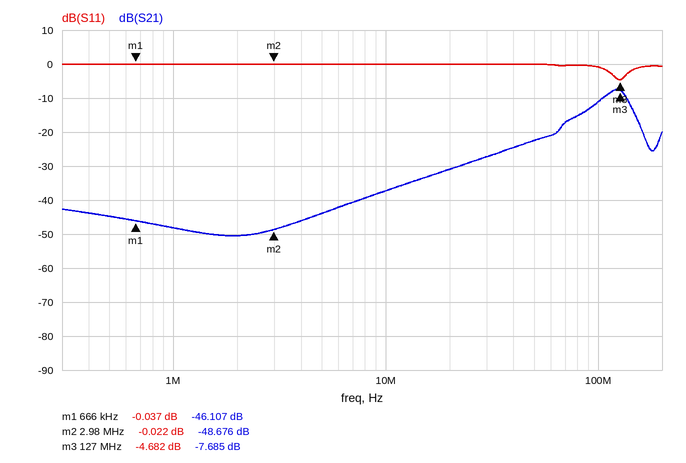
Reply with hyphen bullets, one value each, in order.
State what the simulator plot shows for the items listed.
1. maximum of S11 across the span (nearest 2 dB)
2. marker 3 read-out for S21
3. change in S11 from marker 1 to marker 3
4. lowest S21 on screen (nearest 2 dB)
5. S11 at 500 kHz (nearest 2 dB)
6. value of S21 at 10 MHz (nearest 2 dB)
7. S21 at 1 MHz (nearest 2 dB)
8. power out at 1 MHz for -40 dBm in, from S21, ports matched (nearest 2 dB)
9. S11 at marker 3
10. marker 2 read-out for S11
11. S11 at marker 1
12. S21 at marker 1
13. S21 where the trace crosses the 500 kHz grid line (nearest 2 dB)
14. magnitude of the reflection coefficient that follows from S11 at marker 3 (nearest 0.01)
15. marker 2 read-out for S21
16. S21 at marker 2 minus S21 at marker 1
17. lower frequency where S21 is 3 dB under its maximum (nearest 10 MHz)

- 0 dB
- -7.685 dB
- -4.645 dB
- -50 dB
- 0 dB
- -38 dB
- -48 dB
- -88 dBm
- -4.682 dB
- -0.022 dB
- -0.037 dB
- -46.107 dB
- -44 dB
- 0.58
- -48.676 dB
- -2.569 dB
- 100 MHz
